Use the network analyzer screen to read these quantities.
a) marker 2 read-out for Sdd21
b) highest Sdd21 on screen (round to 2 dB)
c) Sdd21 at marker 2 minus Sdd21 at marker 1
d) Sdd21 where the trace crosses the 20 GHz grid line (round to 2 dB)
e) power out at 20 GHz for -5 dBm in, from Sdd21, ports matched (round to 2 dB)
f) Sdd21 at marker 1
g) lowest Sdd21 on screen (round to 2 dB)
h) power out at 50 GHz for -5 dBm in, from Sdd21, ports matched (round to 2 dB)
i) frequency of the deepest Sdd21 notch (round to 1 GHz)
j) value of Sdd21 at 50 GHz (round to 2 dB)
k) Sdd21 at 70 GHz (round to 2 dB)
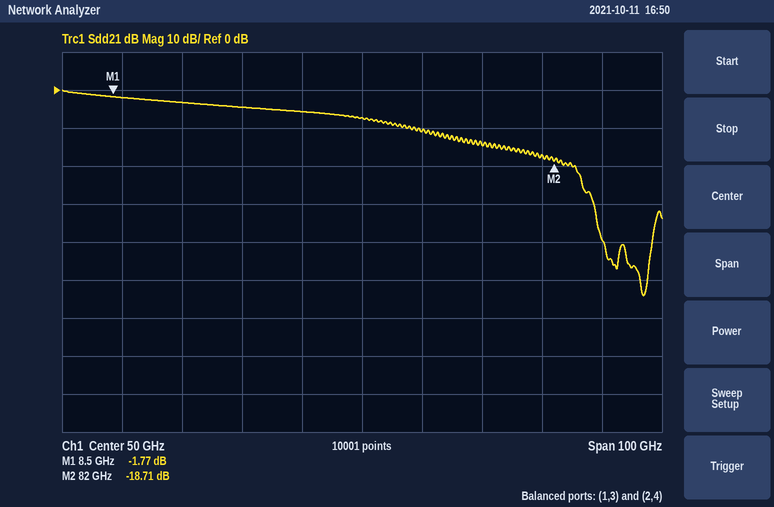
-18.71 dB
0 dB
-16.94 dB
-4 dB
-8 dBm
-1.77 dB
-54 dB
-12 dBm
97 GHz
-8 dB
-14 dB
